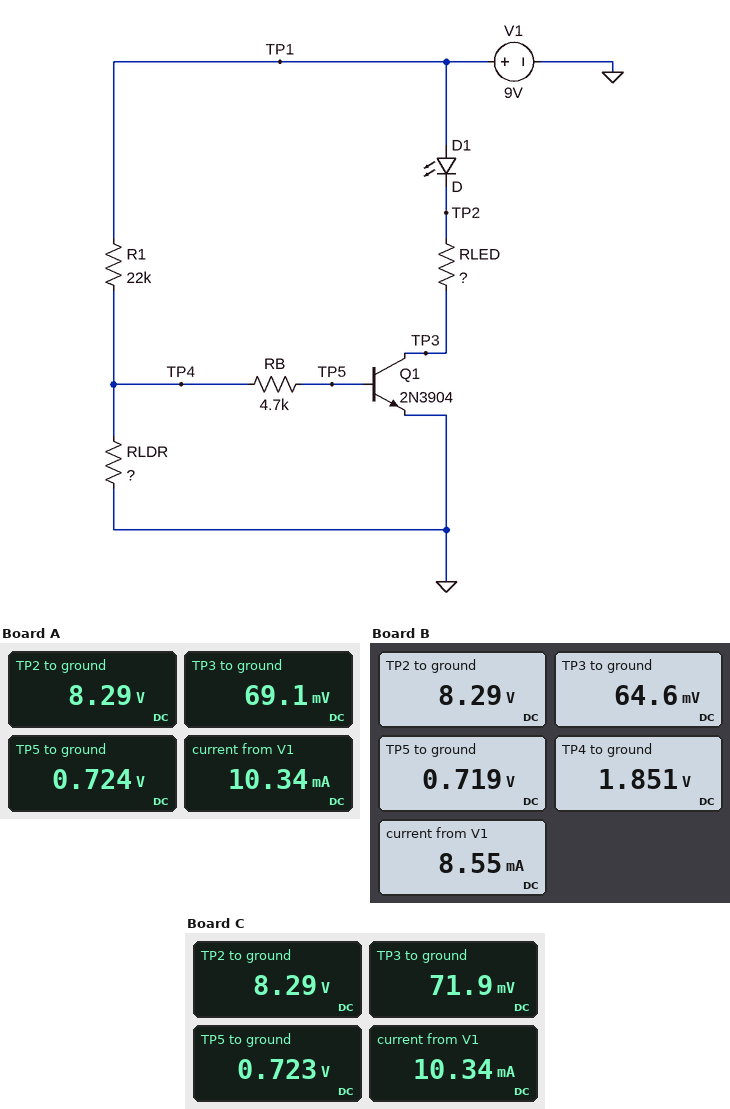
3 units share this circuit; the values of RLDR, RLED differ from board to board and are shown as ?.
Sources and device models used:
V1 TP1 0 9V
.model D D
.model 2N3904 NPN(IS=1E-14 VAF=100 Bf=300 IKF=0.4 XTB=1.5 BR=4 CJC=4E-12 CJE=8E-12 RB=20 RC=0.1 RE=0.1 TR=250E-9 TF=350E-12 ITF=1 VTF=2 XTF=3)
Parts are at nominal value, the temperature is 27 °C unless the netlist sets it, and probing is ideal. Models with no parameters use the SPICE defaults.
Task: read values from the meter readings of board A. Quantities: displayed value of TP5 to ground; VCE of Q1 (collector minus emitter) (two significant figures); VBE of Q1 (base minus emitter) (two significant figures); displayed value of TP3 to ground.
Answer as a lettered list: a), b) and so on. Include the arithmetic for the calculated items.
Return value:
a) 0.724 V
b) 69.1 mV = 69 mV
c) 724 mV = 720 mV
d) 69.1 mV
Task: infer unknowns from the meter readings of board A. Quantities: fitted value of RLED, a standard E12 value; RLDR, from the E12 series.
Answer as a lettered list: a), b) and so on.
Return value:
a) 820 Ω
b) 27 kΩ
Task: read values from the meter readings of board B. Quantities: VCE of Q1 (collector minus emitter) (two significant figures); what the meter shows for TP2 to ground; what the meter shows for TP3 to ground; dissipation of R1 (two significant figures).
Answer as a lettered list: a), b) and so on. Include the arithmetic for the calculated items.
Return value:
a) 64.6 mV = 65 mV
b) 8.29 V
c) 64.6 mV
d) (9 V - 1.851 V)^2 / 22 kΩ = 2.3 mW
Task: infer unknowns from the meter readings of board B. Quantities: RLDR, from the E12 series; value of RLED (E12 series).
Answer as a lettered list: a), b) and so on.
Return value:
a) 22 kΩ
b) 1 kΩ
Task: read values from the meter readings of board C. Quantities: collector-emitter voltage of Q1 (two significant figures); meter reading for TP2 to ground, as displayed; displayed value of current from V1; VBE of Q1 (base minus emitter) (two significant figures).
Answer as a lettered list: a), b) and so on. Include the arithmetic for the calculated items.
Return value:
a) 71.9 mV = 72 mV
b) 8.29 V
c) 10.34 mA
d) 723 mV = 720 mV
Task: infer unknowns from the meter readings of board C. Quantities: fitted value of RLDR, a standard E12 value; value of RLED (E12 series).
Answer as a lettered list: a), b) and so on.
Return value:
a) 18 kΩ
b) 820 Ω
